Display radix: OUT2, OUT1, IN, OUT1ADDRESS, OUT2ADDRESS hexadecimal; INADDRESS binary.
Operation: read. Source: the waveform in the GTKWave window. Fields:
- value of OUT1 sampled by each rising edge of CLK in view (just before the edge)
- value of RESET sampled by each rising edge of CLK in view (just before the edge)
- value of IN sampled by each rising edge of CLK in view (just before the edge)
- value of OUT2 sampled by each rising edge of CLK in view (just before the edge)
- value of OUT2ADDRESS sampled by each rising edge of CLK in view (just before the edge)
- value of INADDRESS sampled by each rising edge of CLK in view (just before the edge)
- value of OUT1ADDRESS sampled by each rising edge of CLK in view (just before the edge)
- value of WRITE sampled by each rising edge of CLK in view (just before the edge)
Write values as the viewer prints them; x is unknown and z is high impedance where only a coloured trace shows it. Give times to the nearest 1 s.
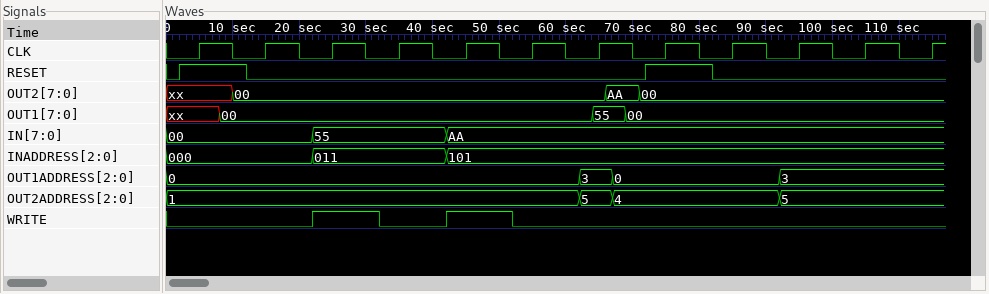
xx, 00, 00, 00, 00, 00, 55, 00, 00, 00, 00, 00
1 0 0 0 0 0 0 1 0 0 0 0
00, 00, 55, 55, AA, AA, AA, AA, AA, AA, AA, AA
xx, 00, 00, 00, 00, 00, 00, 00, 00, 00, 00, 00
1, 1, 1, 1, 1, 1, 5, 4, 4, 5, 5, 5
000, 000, 011, 011, 101, 101, 101, 101, 101, 101, 101, 101
0, 0, 0, 0, 0, 0, 3, 0, 0, 3, 3, 3
0 0 1 0 1 0 0 0 0 0 0 0
